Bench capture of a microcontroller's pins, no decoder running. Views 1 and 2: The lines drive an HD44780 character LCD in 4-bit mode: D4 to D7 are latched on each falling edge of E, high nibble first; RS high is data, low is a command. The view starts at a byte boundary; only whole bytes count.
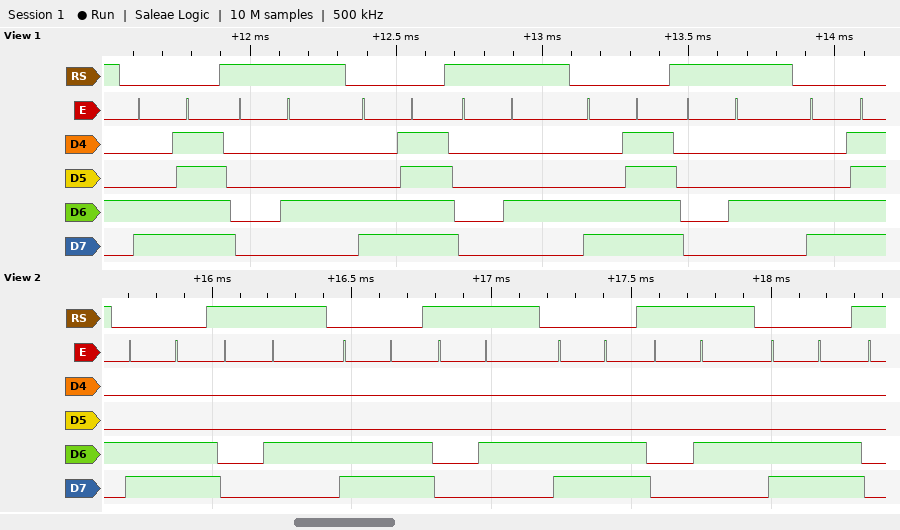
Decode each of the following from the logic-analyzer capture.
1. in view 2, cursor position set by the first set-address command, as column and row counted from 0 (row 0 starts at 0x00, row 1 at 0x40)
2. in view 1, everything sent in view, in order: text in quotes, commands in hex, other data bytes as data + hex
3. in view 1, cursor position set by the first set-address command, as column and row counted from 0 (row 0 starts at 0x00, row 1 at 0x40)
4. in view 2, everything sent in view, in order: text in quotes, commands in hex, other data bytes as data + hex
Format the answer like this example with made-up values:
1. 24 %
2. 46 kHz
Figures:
1. column 12, row 1
2. 0xCF data 04 0xCF data 04 0xCF data 04 0xCF
3. column 15, row 1
4. 0xCC data 04 0xCC data 04 0xCC data 04 0xCC
